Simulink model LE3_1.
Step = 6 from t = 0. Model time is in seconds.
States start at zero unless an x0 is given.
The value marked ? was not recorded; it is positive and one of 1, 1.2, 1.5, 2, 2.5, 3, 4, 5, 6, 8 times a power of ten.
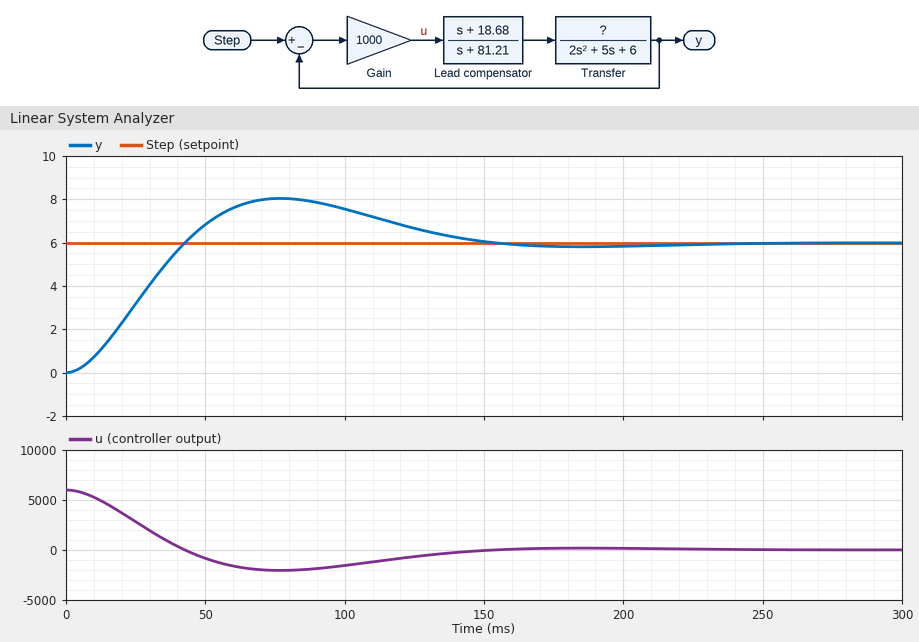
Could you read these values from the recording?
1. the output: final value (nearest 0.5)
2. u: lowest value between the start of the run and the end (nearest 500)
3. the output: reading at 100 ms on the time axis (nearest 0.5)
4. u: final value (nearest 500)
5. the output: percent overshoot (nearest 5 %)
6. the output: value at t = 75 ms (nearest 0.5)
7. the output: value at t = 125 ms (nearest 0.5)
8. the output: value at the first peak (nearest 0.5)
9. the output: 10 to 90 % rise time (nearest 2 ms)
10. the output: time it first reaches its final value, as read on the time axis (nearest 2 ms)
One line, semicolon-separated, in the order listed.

6.0; -2000; 7.5; 0; 35 %; 8.0; 6.5; 8.0; 30 ms; 42 ms
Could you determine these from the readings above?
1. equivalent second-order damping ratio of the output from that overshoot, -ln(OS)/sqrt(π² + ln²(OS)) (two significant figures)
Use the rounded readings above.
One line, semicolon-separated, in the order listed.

0.32
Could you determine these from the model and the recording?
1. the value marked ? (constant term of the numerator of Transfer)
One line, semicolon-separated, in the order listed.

6
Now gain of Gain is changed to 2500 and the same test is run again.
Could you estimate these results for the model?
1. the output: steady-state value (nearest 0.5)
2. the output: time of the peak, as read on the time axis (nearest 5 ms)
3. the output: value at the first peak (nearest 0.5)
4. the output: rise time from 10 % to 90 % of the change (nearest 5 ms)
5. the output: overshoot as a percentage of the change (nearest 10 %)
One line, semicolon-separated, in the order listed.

6.0; 40 ms; 8.5; 15 ms; 40 %
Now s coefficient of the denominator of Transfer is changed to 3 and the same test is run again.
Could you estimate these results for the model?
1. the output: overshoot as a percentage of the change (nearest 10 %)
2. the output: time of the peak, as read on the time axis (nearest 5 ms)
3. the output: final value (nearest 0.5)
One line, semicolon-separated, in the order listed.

40 %; 75 ms; 6.0
